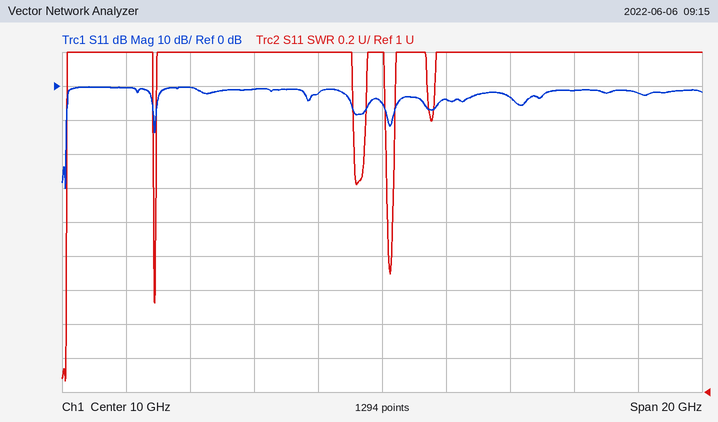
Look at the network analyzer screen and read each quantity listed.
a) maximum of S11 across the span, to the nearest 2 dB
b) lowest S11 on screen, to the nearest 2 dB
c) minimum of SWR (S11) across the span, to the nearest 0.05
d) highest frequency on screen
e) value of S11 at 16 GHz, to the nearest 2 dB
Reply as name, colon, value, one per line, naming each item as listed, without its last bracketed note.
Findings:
maximum of S11 across the span, to the nearest 2 dB: 0 dB
lowest S11 on screen, to the nearest 2 dB: -30 dB
minimum of SWR (S11) across the span, to the nearest 0.05: 1.05
highest frequency on screen: 20 GHz
value of S11 at 16 GHz, to the nearest 2 dB: -2 dB
